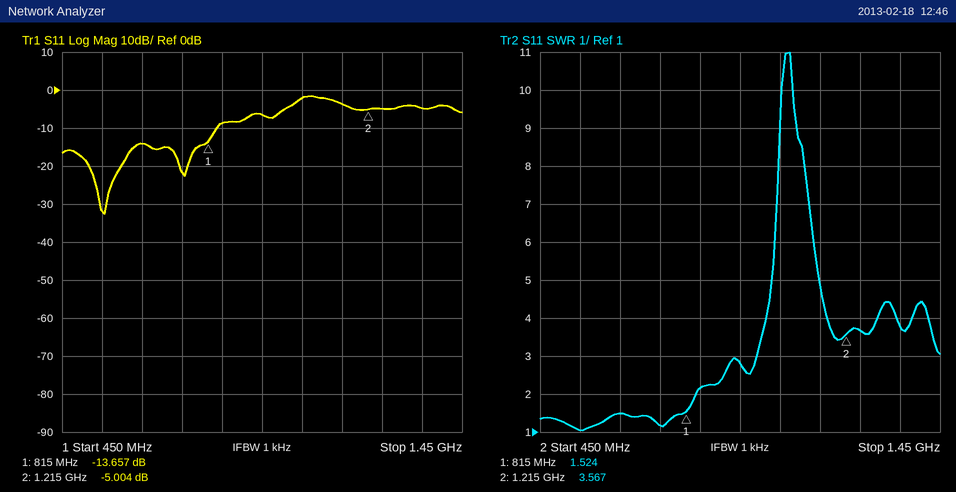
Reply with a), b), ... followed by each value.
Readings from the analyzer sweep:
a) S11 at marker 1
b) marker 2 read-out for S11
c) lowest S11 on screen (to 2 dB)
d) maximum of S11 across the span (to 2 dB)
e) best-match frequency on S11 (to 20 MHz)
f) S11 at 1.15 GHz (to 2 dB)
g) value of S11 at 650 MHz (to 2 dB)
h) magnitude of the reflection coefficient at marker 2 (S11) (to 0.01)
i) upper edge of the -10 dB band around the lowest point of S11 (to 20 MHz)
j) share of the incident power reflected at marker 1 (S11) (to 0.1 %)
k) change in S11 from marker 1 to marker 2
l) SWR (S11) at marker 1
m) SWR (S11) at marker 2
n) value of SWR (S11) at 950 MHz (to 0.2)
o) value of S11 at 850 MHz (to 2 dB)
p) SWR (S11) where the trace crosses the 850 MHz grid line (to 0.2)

a) -13.657 dB
b) -5.004 dB
c) -32 dB
d) -2 dB
e) 560 MHz
f) -4 dB
g) -14 dB
h) 0.56
i) 840 MHz
j) 4.3 %
k) 8.653 dB
l) 1.524
m) 3.567
n) 2.8
o) -8 dB
p) 2.2
